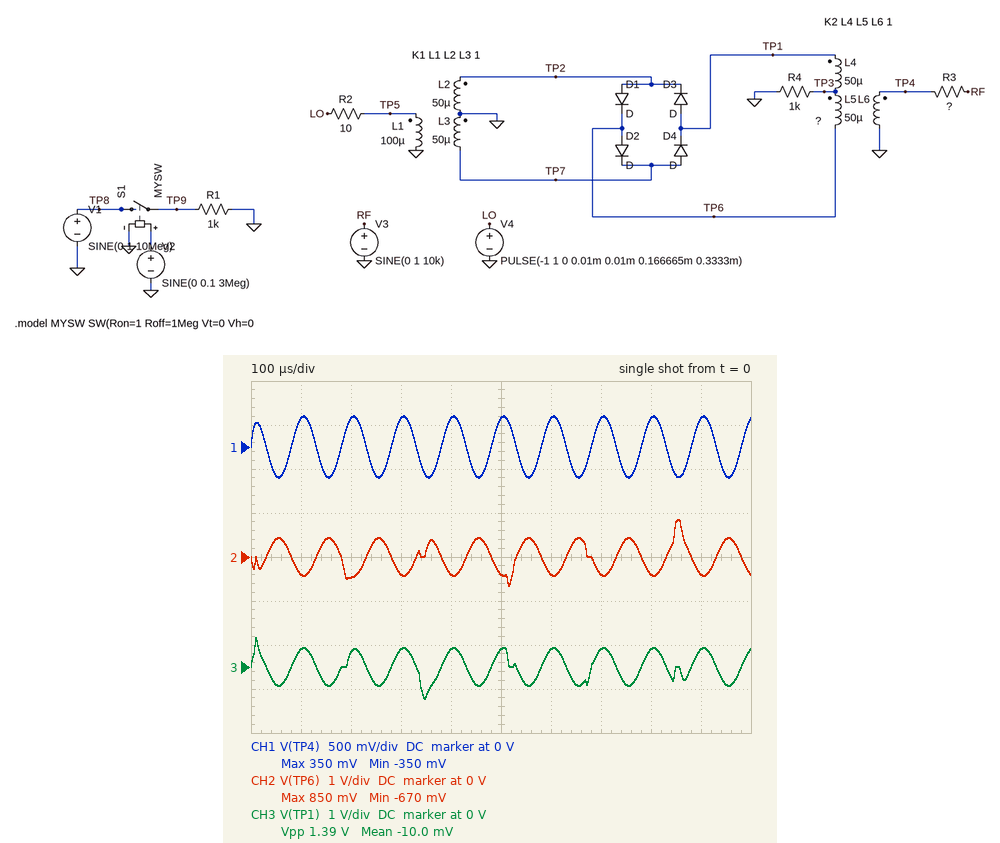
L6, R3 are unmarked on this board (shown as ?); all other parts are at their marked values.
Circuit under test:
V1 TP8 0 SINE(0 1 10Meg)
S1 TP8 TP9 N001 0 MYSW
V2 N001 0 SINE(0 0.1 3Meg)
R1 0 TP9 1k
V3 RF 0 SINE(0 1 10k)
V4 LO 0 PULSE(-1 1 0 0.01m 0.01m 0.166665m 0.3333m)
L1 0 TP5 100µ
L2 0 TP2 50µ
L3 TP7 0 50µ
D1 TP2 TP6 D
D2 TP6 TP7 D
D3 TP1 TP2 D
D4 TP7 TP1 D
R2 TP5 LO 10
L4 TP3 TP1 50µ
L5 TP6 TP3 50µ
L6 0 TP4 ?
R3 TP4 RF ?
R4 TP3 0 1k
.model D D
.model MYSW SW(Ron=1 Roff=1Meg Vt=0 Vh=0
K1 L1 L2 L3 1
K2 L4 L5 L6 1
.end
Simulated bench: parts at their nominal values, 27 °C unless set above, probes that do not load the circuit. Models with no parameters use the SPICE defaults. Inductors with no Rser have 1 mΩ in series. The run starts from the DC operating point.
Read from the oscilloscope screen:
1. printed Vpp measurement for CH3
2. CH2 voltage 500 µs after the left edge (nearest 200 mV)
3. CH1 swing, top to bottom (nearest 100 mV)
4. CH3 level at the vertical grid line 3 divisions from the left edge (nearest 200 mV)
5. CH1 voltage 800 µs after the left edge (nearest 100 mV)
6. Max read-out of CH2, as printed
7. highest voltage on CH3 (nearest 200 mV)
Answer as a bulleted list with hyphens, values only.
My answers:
- 1.39 V
- -400 mV
- 700 mV
- 400 mV
- 300 mV
- 850 mV
- 600 mV
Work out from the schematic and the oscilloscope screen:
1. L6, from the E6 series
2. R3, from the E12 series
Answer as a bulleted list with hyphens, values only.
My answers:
- 33 µH
- 5.6 Ω
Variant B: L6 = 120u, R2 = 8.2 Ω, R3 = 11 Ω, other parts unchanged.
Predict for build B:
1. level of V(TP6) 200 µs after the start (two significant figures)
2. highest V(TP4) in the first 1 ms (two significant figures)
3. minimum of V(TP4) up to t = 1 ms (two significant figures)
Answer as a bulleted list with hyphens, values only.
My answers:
- -370 mV
- 570 mV
- -570 mV
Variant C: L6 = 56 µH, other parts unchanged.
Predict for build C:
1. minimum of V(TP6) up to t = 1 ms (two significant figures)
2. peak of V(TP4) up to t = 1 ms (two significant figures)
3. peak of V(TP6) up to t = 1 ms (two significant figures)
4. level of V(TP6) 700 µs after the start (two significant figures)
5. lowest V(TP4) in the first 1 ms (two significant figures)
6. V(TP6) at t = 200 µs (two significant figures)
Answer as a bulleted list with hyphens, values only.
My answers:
- -890 mV
- 530 mV
- 990 mV
- -420 mV
- -530 mV
- -510 mV
